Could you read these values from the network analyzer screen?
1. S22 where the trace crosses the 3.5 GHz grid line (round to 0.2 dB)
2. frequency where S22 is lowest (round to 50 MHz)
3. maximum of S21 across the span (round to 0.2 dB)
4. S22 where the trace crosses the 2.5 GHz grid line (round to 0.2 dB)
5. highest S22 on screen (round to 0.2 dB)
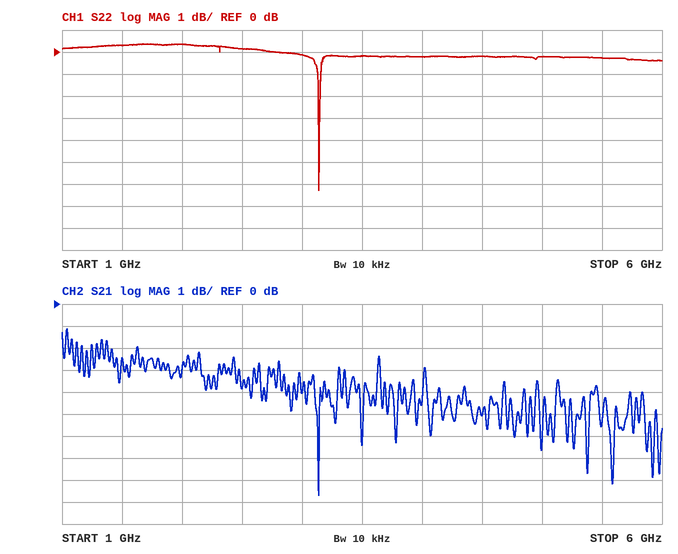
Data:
-0.2 dB
3.15 GHz
-1.2 dB
0.2 dB
0.4 dB
